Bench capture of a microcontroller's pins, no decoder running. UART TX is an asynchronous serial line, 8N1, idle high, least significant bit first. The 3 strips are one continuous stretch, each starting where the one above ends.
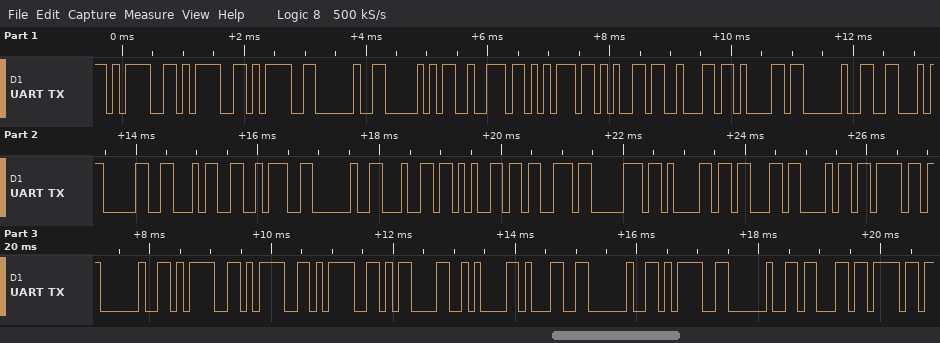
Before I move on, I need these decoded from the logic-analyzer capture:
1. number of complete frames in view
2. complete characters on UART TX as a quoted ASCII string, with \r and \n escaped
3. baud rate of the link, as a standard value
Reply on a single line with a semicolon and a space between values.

36; "=== Prueba F04: despacho ===\r\n1 = co"; 9600 baud
